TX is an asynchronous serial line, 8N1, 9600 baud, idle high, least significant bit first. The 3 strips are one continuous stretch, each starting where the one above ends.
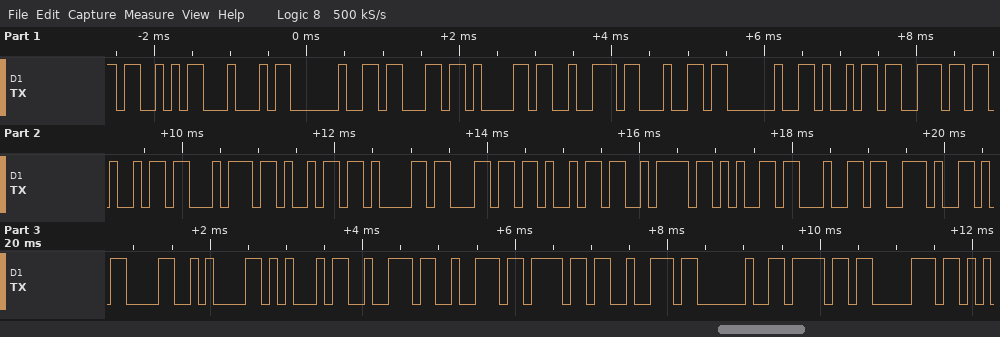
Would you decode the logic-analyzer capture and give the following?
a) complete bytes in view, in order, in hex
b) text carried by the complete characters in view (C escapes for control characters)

0x53 0x44 0x20 0x63 0x61 0x72 0x64 0x20 0x69 0x6E 0x69 0x74 0x69 0x61 0x6C 0x69 0x7A 0x65 0x64 0x2E 0x0D 0x0A 0x45 0x72 0x72 0x6F 0x72 0x20 0x6F 0x70
"SD card initialized.\r\nError op"
